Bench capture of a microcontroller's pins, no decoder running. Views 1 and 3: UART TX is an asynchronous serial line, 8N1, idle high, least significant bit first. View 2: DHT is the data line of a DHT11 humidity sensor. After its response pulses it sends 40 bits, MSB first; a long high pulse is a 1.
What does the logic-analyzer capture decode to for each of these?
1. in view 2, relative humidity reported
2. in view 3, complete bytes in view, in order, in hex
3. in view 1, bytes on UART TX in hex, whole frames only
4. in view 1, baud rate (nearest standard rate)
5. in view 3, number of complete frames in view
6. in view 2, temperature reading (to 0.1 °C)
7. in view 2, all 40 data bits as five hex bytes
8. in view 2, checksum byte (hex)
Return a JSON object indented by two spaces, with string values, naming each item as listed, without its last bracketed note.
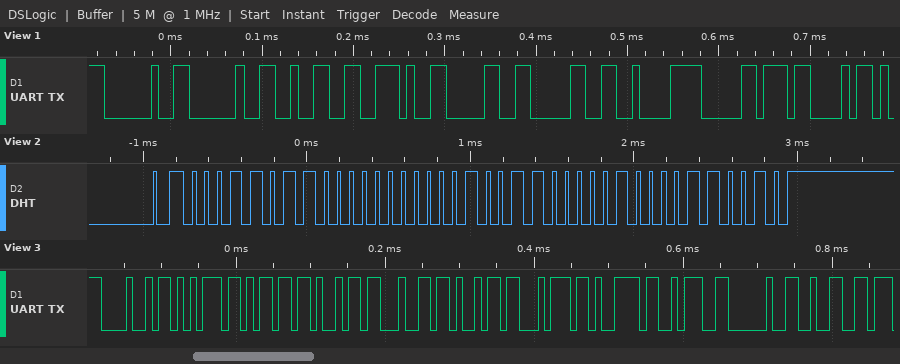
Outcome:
{
  "in view 2, relative humidity reported": "27 %",
  "in view 3, complete bytes in view, in order, in hex": "48 75 6D 69 64 69 74 79 3A 20 32",
  "in view 1, bytes on UART TX in hex, whole frames only": "20 20 32 2E 30 30 C2 B0 43",
  "in view 1, baud rate": "115200 baud",
  "in view 3, number of complete frames in view": "11",
  "in view 2, temperature reading": "19.4 °C",
  "in view 2, all 40 data bits as five hex bytes": "1B 00 13 04 32",
  "in view 2, checksum byte": "0x32"
}
